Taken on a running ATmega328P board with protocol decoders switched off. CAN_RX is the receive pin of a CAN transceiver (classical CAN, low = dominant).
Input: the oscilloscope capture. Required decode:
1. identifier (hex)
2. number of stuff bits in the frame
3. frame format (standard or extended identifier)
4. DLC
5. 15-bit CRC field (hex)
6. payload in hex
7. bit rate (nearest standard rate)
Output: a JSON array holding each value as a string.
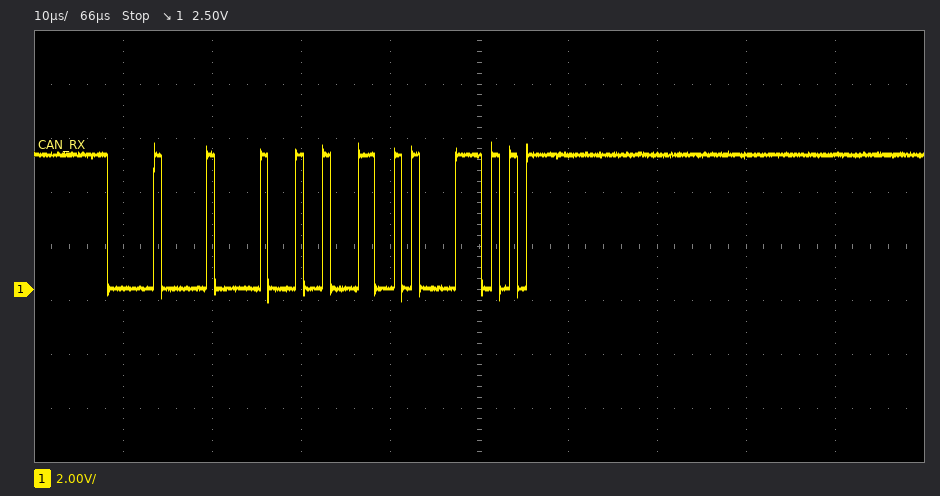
["0x000", "3", "standard", "1", "0x143A", "23", "1000 kbit/s"]
